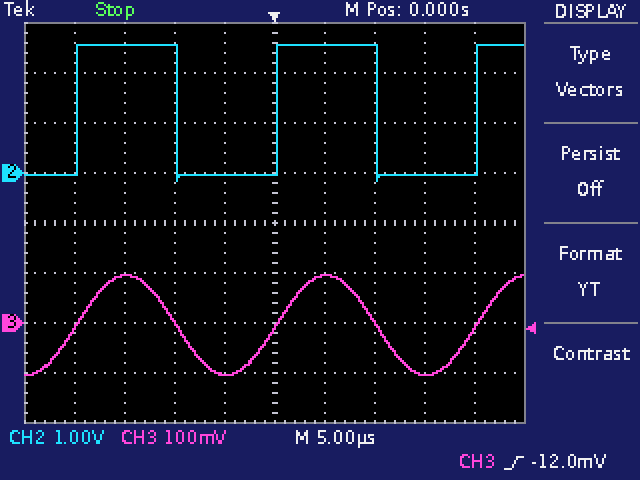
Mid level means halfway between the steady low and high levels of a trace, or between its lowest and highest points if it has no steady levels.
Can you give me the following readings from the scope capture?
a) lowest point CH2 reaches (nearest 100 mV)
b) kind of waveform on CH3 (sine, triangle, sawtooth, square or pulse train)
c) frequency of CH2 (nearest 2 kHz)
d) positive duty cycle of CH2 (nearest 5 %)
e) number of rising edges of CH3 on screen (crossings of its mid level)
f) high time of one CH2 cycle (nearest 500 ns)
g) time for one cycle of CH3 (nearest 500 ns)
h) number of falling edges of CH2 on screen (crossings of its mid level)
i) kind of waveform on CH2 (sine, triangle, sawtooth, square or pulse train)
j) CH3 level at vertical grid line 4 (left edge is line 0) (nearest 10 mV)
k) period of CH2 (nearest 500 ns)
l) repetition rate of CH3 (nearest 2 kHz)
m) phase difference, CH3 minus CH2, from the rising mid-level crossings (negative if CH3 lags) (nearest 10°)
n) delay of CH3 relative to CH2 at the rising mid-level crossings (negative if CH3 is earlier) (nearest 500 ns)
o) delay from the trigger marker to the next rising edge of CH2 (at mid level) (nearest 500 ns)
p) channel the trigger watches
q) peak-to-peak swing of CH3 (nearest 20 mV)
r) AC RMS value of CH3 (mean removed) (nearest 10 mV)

-200 mV
sine
50 kHz
50 %
3
10.0 µs
20.0 µs
2
square
-100 mV
20.0 µs
50 kHz
0°
0.0 µs
500 ns
CH3
200 mV
70 mV
